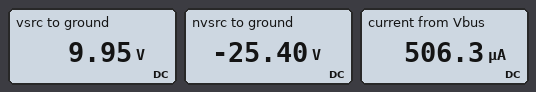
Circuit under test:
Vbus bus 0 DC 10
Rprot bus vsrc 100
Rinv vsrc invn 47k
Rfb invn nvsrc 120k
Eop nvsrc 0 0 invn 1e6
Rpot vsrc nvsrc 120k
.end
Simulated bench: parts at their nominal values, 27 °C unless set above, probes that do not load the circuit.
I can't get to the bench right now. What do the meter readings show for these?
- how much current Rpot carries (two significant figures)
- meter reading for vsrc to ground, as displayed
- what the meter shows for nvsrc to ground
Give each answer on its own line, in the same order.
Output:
290 µA
9.95 V
-25.40 V
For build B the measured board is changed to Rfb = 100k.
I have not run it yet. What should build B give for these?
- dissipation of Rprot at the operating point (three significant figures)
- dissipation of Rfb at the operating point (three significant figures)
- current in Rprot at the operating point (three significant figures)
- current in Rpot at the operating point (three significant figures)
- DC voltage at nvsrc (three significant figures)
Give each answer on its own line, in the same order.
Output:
22.2 µW
4.48 mW
471 µA
259 µA
-21.2 V
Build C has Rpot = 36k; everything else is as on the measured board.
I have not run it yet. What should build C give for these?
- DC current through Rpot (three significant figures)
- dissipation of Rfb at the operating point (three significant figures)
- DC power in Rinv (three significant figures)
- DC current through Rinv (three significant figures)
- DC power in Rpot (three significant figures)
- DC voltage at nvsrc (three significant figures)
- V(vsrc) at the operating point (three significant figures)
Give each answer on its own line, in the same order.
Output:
975 µA
5.30 mW
2.08 mW
210 µA
34.2 mW
-25.2 V
9.88 V
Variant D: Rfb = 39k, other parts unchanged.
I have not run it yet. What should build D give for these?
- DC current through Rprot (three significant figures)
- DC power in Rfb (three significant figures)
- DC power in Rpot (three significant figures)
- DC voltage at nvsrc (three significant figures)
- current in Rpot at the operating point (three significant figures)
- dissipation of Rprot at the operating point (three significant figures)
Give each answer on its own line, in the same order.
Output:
364 µA
1.75 mW
2.77 mW
-8.27 V
152 µA
13.2 µW
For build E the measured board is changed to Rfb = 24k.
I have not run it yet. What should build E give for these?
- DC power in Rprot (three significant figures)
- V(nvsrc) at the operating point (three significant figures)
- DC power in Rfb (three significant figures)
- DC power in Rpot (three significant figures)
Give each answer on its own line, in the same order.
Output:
11.4 µW
-5.09 V
1.08 mW
1.89 mW
